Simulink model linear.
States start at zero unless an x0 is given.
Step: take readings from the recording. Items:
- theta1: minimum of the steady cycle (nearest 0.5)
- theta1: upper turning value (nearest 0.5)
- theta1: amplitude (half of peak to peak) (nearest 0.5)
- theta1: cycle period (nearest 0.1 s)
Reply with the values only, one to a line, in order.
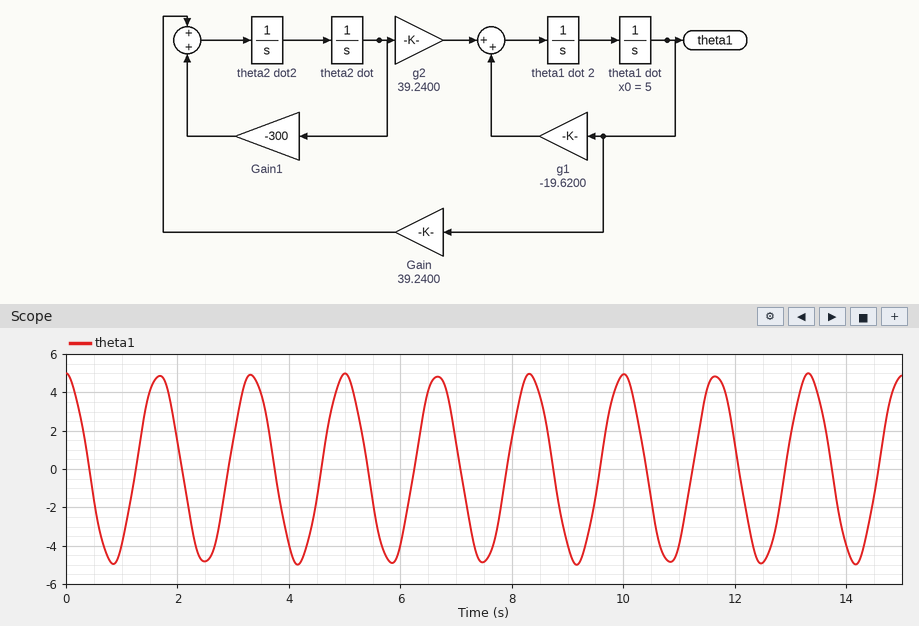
-5.0
5.0
5.0
1.7 s
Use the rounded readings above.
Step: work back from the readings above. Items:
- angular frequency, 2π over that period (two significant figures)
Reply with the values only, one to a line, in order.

3.7 rad/s
